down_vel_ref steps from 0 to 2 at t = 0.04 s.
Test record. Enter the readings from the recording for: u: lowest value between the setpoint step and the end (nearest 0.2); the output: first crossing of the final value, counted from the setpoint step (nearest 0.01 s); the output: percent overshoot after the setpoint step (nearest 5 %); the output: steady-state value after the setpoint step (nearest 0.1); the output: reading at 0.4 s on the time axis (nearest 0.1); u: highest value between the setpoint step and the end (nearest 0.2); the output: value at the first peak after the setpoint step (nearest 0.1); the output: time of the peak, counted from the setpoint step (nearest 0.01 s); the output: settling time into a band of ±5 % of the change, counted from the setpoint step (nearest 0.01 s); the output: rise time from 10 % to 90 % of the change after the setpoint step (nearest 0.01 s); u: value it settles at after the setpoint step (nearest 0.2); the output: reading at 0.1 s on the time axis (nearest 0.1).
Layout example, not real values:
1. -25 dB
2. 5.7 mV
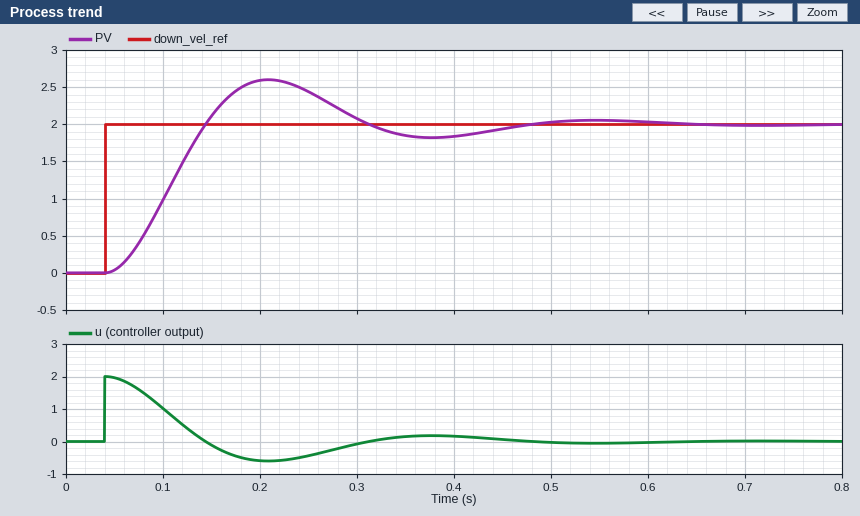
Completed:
1. -0.6
2. 0.10 s
3. 30 %
4. 2.0
5. 1.8
6. 2.0
7. 2.6
8. 0.17 s
9. 0.39 s
10. 0.07 s
11. 0.0
12. 1.0
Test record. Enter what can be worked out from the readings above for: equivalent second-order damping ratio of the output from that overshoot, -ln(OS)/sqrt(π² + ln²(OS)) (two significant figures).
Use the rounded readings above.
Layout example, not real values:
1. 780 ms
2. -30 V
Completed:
1. 0.36
